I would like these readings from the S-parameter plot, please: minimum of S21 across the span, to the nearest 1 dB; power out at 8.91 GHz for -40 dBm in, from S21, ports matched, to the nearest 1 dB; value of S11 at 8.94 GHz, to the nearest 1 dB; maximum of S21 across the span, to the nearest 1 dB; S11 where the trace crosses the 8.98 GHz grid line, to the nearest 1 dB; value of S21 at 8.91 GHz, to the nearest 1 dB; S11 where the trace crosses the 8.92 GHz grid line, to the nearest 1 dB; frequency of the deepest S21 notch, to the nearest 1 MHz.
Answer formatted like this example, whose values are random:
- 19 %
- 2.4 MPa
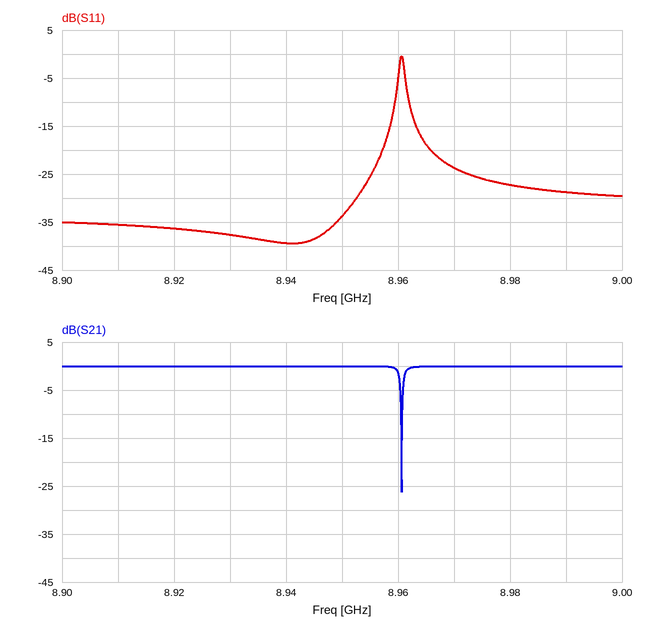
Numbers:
- -26 dB
- -40 dBm
- -39 dB
- 0 dB
- -27 dB
- 0 dB
- -36 dB
- 8.961 GHz
